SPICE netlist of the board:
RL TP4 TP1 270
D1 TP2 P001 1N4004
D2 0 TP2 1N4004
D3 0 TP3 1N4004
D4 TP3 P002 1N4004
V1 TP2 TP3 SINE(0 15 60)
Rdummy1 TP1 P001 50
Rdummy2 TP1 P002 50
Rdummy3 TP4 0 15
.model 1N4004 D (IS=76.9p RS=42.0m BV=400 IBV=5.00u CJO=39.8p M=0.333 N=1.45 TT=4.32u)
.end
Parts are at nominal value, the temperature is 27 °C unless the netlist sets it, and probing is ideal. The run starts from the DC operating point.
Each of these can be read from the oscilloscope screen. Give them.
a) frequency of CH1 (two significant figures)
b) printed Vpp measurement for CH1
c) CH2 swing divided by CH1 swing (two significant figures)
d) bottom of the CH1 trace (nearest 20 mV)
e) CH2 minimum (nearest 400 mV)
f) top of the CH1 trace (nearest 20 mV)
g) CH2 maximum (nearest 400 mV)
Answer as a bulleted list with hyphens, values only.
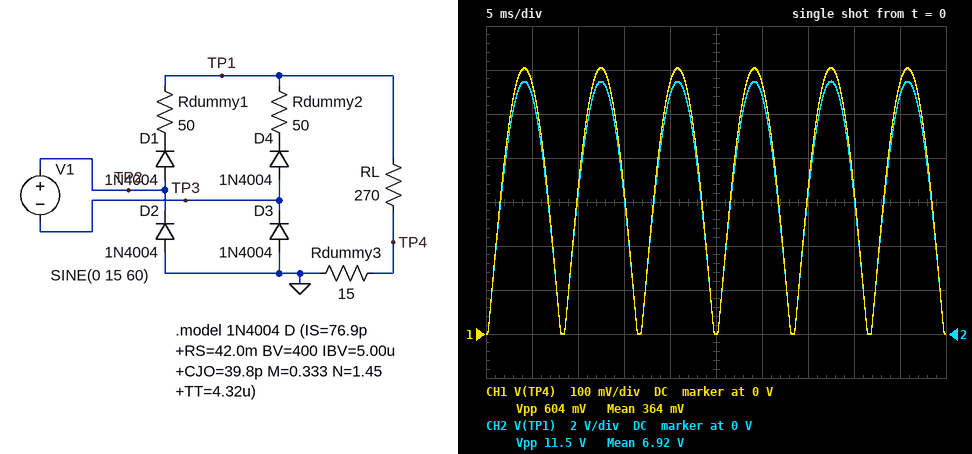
- 120 Hz
- 604 mV
- 19
- 0 V
- 0 V
- 600 mV
- 11.6 V
